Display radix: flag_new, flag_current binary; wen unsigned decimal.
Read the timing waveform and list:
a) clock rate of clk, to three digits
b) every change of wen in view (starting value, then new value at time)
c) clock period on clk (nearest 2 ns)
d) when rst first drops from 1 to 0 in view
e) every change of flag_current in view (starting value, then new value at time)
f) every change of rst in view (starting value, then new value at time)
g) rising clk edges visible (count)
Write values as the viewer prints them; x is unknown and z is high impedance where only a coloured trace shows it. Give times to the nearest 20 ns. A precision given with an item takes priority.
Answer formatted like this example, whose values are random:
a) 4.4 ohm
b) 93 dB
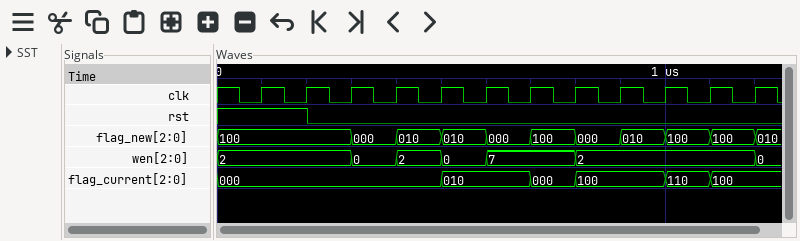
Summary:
a) 10.0 MHz
b) 2, 0 at 300 ns, 2 at 400 ns, 0 at 500 ns, 7 at 600 ns, 2 at 800 ns, 0 at 1200 ns
c) 100 ns
d) 200 ns
e) 000, 010 at 500 ns, 000 at 700 ns, 100 at 800 ns, 110 at 1000 ns, 100 at 1100 ns
f) 1, 0 at 200 ns
g) 12
